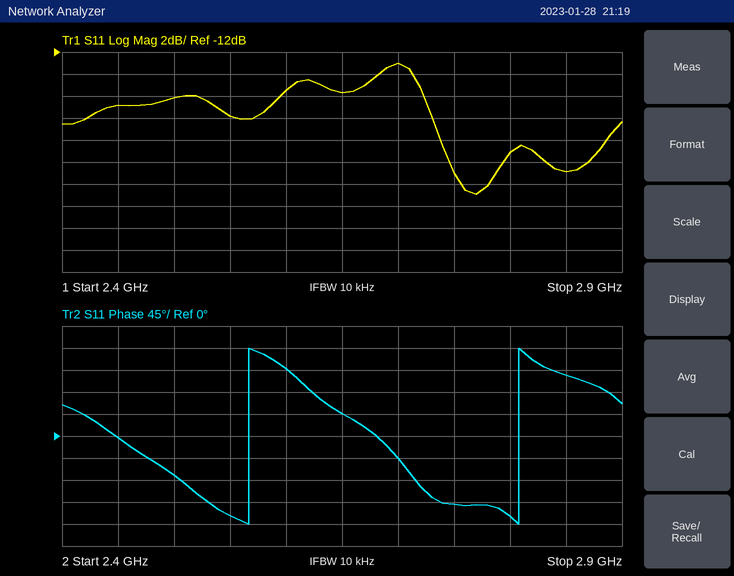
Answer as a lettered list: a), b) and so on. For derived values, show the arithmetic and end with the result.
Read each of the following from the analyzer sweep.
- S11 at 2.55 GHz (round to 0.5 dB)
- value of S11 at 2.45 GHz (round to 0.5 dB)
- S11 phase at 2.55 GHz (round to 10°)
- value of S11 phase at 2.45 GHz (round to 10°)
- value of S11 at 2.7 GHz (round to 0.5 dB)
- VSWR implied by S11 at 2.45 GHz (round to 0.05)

a) -18.0 dB
b) -17.0 dB
c) -160°
d) 0°
e) -13.0 dB
f) |Γ| = 10^(-17/20) = 0.1413; VSWR = (1 + 0.1413)/(1 − 0.1413) ≈ 1.33, so 1.35 to the nearest 0.05
